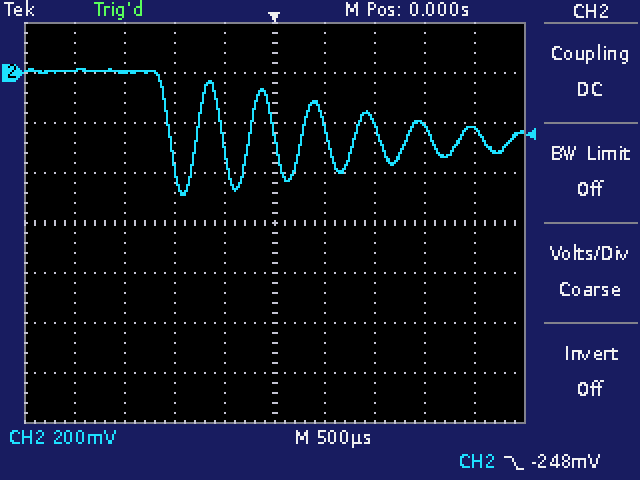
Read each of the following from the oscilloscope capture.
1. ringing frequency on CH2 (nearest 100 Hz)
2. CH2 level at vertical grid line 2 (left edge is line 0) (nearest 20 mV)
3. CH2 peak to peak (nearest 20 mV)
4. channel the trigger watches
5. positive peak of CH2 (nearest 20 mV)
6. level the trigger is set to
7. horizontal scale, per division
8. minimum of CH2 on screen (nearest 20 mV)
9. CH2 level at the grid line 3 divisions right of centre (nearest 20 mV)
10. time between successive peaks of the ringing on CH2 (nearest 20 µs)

1.9 kHz
0 mV
500 mV
CH2
20 mV
-248 mV
500 µs
-480 mV
-220 mV
520 µs
